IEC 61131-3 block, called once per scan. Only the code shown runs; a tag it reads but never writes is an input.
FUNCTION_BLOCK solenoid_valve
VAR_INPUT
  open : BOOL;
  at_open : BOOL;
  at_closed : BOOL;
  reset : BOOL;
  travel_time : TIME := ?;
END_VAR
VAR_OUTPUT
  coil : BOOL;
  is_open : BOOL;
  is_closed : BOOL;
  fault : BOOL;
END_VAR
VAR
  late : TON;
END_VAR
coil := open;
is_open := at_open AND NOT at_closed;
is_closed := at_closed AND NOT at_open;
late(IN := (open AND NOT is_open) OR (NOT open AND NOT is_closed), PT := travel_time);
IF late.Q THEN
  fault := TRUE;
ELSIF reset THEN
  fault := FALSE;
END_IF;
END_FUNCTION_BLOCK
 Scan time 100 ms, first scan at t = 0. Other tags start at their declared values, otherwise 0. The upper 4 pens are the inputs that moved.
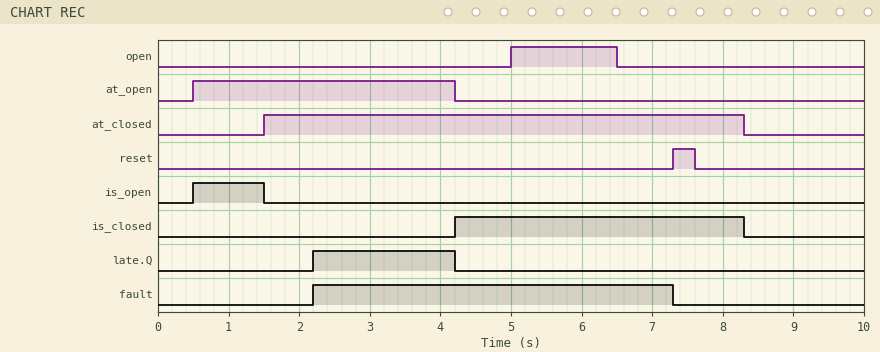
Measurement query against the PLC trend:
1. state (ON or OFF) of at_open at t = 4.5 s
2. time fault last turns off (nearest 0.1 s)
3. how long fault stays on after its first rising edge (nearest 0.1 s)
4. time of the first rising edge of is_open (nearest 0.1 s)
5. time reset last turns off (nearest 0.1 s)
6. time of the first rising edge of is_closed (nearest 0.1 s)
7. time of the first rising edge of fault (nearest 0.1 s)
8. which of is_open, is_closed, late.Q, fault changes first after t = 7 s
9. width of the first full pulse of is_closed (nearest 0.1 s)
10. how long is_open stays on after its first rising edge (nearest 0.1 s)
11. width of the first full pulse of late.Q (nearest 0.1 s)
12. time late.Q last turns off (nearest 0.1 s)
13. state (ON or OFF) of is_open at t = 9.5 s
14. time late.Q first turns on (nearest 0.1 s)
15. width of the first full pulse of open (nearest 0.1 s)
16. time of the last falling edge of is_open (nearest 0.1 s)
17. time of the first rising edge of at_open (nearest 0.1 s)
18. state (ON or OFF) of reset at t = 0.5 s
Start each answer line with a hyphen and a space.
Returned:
- OFF
- 7.3 s
- 5.1 s
- 0.5 s
- 7.6 s
- 4.2 s
- 2.2 s
- fault
- 4.1 s
- 1.0 s
- 2.0 s
- 4.2 s
- OFF
- 2.2 s
- 1.5 s
- 1.5 s
- 0.5 s
- OFF
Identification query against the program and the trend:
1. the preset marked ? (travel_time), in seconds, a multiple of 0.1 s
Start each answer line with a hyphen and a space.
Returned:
- 2.2 s
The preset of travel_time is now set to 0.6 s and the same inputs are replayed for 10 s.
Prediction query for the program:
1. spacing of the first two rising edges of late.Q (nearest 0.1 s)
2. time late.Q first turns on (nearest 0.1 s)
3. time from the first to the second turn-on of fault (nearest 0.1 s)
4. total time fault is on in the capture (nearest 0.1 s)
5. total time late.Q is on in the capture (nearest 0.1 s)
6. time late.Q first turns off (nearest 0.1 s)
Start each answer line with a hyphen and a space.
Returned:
- 5.0 s
- 0.6 s
- 8.3 s
- 7.8 s
- 5.6 s
- 4.2 s
